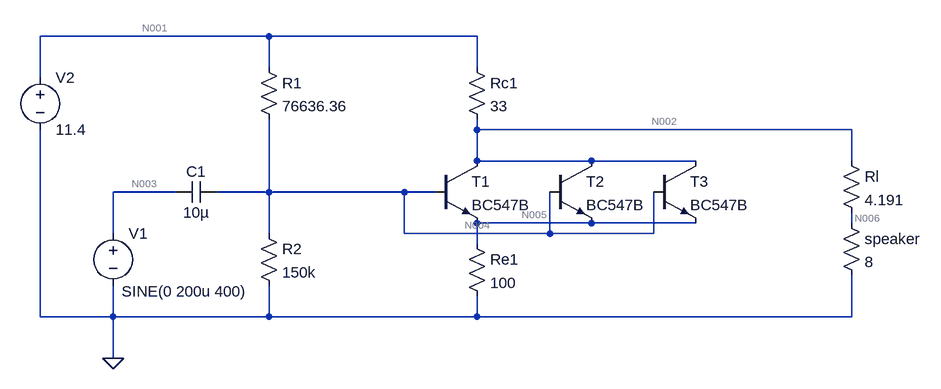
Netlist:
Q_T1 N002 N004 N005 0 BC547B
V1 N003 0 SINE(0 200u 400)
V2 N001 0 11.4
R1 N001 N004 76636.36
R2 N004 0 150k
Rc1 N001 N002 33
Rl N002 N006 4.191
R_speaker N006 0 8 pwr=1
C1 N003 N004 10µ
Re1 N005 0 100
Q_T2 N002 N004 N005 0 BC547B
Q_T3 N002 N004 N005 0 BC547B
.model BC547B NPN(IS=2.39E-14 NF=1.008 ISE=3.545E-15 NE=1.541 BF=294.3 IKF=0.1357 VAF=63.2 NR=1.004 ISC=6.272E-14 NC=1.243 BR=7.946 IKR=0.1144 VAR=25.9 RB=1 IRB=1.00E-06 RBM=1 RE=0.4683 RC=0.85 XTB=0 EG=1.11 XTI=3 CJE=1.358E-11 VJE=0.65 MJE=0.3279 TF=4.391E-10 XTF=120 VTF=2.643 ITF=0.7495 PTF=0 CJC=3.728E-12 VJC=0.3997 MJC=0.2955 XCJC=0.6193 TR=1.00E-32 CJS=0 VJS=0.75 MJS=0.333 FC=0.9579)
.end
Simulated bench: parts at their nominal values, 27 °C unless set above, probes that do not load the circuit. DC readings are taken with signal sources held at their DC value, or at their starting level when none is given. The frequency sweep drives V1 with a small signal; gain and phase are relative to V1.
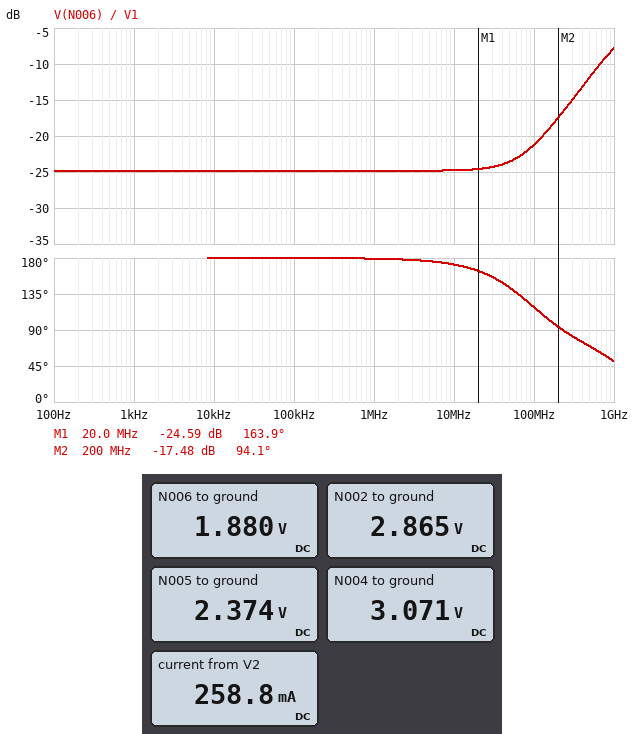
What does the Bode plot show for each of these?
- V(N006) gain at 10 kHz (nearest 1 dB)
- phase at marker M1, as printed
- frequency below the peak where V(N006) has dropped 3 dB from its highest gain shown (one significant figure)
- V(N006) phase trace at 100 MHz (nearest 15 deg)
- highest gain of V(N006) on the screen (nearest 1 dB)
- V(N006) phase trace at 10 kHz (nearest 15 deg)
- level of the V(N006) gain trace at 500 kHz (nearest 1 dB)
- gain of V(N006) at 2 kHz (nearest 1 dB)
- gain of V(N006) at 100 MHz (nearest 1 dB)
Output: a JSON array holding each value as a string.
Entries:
["-25 dB", "163.9 deg", "600 MHz", "120 deg", "-8 dB", "180 deg", "-25 dB", "-25 dB", "-21 dB"]
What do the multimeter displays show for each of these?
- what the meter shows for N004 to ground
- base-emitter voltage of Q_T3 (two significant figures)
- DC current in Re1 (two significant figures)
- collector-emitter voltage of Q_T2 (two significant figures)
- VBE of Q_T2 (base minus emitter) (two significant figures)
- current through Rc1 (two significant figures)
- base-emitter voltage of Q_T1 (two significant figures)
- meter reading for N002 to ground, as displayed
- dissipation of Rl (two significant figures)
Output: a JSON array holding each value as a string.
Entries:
["3.071 V", "700 mV", "24 mA", "490 mV", "700 mV", "260 mA", "700 mV", "2.865 V", "230 mW"]
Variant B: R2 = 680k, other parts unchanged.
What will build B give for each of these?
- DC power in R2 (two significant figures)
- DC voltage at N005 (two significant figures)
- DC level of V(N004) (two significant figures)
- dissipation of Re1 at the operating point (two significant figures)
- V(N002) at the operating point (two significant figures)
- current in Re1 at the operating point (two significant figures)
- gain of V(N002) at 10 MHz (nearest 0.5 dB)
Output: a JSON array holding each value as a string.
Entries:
["16 µW", "2.6 V", "3.3 V", "69 mW", "2.8 V", "26 mA", "-20.0 dB"]
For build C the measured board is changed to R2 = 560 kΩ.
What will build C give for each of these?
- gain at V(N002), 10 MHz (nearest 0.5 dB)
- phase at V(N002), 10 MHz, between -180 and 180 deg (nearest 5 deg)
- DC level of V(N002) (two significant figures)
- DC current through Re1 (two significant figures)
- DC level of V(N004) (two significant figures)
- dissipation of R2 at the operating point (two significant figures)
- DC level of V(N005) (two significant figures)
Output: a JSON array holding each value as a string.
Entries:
["-20.0 dB", "150 deg", "2.8 V", "26 mA", "3.3 V", "20 µW", "2.6 V"]
